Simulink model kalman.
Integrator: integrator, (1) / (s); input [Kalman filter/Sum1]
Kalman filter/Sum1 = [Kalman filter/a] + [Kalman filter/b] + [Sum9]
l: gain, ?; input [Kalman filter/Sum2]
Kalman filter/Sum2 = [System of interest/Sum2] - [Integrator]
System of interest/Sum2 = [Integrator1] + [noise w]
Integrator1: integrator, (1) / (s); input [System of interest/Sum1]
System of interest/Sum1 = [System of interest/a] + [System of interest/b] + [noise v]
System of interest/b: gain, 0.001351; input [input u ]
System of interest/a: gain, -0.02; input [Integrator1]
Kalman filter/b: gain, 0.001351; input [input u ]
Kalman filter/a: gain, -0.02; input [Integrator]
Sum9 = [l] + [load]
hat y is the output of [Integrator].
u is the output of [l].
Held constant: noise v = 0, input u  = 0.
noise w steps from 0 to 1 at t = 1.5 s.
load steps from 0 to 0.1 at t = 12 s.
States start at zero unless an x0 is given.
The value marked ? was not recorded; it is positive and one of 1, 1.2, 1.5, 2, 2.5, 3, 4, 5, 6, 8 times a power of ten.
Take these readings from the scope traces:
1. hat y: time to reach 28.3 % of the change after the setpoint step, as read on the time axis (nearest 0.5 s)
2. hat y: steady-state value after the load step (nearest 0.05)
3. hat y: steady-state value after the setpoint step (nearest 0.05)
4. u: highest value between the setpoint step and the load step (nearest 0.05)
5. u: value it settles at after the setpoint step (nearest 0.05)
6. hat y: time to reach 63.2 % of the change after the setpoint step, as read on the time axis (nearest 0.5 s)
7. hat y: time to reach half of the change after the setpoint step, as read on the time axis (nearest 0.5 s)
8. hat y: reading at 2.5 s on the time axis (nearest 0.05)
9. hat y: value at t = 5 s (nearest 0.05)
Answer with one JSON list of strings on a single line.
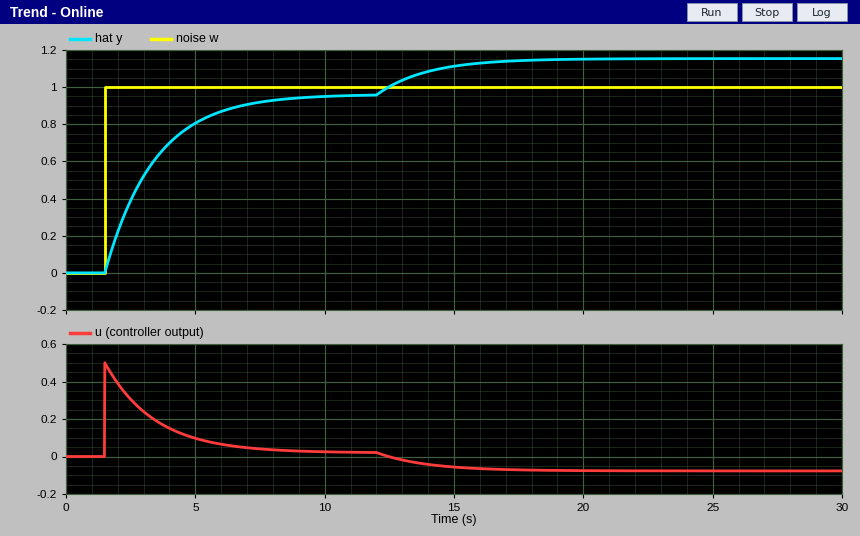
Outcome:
["2.0 s", "1.15", "0.95", "0.50", "0.00", "3.5 s", "3.0 s", "0.40", "0.80"]
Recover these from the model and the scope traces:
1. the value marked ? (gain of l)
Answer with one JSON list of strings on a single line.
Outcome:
["0.5"]
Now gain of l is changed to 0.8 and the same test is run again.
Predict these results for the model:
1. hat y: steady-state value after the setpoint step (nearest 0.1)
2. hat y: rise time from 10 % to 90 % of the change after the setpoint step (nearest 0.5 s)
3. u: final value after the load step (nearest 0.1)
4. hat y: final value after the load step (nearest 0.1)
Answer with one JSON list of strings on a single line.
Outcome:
["1.0", "2.5 s", "-0.1", "1.1"]
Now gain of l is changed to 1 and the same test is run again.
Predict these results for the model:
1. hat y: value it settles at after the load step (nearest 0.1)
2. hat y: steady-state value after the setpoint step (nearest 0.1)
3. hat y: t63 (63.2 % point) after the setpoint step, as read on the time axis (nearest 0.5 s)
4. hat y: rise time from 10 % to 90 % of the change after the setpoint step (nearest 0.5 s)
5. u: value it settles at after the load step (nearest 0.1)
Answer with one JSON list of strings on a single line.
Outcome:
["1.1", "1.0", "2.5 s", "2.0 s", "-0.1"]
